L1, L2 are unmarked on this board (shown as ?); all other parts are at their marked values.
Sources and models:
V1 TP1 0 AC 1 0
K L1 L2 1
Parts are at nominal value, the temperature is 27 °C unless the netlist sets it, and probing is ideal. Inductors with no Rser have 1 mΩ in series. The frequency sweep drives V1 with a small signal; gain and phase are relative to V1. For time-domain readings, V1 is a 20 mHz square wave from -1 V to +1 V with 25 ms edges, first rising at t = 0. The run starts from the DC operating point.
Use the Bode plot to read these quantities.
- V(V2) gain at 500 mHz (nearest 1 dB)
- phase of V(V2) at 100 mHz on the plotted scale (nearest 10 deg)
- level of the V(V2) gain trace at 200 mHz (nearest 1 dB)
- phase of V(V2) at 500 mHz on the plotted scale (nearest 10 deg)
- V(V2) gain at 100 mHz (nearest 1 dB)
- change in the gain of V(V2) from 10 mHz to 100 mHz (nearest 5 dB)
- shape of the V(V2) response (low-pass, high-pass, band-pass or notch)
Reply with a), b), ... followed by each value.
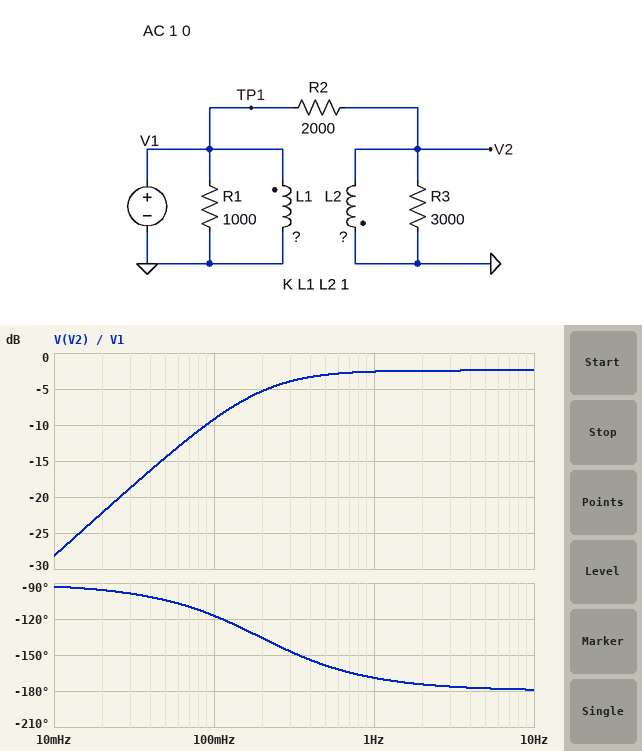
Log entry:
a) -3 dB
b) -120 deg
c) -5 dB
d) -160 deg
e) -9 dB
f) 20 dB
g) high-pass
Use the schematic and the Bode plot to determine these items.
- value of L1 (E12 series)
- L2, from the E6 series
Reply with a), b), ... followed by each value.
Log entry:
a) 820 µH
b) 470 µH
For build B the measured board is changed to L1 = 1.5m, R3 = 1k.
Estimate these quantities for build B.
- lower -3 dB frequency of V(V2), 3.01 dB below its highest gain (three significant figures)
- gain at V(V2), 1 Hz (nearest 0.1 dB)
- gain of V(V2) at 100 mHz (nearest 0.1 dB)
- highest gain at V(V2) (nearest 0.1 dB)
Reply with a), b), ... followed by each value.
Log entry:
a) 106 mHz
b) -5.1 dB
c) -8.3 dB
d) -5.0 dB
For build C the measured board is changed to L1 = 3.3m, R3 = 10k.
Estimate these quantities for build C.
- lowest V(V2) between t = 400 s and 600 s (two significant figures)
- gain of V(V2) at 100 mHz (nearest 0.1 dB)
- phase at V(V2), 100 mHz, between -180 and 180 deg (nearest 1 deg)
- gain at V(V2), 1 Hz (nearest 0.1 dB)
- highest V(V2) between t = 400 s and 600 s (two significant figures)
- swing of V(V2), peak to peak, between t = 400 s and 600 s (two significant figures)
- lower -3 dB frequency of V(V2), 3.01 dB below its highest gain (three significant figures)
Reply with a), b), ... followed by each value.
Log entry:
a) -750 mV
b) -9.4 dB
c) -154 deg
d) -8.5 dB
e) 750 mV
f) 1.5 V
g) 48.2 mHz
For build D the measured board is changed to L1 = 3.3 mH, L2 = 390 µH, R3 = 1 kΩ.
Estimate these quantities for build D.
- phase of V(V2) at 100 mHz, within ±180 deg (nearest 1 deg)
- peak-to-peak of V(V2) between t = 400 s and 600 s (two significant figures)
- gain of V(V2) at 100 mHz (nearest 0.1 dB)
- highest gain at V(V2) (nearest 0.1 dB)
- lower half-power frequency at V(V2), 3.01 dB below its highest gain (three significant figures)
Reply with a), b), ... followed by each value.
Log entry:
a) -154 deg
b) 1.4 V
c) -10.2 dB
d) -9.3 dB
e) 48.2 mHz
